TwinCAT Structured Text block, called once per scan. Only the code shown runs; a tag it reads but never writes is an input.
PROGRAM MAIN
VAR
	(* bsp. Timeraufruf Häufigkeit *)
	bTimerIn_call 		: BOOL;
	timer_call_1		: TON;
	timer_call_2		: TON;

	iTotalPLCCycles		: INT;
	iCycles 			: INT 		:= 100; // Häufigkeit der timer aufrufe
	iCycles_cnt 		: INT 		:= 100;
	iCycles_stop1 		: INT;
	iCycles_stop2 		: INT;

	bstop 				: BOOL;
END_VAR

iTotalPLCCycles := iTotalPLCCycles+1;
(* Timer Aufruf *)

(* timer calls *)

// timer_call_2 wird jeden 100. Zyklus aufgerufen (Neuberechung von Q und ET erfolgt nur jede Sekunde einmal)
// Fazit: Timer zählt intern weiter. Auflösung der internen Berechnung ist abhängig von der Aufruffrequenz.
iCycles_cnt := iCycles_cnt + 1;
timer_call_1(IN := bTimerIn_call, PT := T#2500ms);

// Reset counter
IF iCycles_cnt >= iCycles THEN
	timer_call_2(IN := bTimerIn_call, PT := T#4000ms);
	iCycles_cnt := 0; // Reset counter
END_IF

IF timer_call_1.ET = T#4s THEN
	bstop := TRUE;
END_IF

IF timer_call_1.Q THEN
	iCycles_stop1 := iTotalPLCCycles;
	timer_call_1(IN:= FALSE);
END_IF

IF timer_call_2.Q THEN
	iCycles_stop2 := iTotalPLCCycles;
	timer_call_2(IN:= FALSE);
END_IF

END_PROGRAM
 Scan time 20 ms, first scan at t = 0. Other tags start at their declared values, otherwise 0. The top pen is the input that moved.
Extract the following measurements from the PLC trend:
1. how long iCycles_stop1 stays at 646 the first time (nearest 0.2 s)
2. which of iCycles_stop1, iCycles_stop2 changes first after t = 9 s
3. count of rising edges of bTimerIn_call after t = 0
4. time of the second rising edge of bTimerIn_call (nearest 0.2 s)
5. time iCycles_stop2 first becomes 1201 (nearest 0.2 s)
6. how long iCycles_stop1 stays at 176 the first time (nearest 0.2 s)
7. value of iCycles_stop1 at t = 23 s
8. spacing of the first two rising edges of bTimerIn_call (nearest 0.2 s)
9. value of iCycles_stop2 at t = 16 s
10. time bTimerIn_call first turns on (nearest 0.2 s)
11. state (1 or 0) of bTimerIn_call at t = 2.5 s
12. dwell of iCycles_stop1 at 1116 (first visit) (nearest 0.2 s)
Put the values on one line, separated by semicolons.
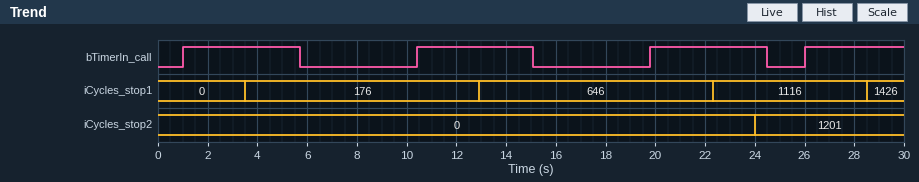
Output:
9.4 s; iCycles_stop1; 4; 10.4 s; 24.0 s; 9.4 s; 1116; 9.4 s; 0; 1.0 s; 1; 6.2 s
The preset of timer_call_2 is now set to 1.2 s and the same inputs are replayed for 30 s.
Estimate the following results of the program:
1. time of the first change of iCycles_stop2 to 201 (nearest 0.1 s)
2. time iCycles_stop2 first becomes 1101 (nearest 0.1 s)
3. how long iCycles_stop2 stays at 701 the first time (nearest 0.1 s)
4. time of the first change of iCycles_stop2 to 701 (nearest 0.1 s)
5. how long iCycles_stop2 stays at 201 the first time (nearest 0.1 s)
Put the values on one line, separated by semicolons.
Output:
4.0 s; 22.0 s; 8.0 s; 14.0 s; 10.0 s
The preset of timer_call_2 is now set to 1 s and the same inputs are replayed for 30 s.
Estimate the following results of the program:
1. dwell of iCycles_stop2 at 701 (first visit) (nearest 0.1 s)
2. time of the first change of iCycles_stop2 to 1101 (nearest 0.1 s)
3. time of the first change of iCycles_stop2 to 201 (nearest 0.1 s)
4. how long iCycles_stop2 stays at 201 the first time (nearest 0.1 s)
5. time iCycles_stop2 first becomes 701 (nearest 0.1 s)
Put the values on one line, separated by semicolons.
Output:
8.0 s; 22.0 s; 4.0 s; 10.0 s; 14.0 s
